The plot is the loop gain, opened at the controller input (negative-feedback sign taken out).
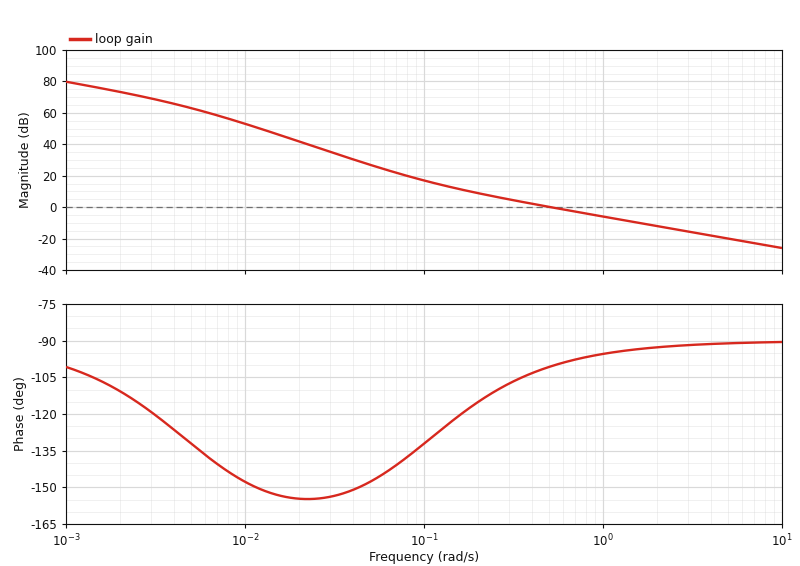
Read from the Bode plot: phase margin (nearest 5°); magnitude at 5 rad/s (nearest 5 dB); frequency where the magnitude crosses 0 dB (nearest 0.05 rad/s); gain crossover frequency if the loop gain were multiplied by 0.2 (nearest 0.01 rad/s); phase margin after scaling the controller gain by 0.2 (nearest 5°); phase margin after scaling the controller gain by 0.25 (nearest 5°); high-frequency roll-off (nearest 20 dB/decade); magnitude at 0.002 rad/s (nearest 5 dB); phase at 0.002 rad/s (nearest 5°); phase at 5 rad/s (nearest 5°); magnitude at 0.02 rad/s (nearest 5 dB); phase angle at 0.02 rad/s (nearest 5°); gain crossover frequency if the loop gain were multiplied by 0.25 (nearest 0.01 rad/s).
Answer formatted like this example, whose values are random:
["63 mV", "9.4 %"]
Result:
["80°", "-20 dB", "0.50 rad/s", "0.13 rad/s", "55°", "60°", "-20 dB/decade", "75 dB", "-110°", "-90°", "40 dB", "-155°", "0.15 rad/s"]
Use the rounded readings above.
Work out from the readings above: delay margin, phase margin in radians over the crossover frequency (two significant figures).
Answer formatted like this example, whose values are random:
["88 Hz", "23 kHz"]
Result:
["2.8 s"]
